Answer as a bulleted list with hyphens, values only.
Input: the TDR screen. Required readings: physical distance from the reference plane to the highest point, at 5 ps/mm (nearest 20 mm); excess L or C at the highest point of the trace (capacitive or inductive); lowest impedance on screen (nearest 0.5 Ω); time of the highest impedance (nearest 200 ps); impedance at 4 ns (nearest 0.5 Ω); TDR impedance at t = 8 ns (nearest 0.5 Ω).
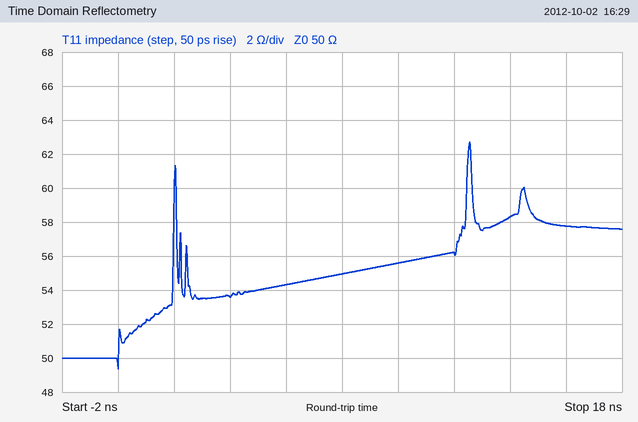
- 1.26 m
- inductive
- 49.5 Ω
- 12.6 ns
- 53.5 Ω
- 55.0 Ω
